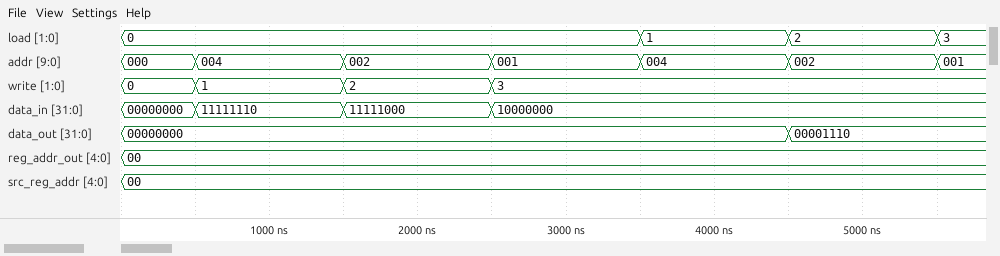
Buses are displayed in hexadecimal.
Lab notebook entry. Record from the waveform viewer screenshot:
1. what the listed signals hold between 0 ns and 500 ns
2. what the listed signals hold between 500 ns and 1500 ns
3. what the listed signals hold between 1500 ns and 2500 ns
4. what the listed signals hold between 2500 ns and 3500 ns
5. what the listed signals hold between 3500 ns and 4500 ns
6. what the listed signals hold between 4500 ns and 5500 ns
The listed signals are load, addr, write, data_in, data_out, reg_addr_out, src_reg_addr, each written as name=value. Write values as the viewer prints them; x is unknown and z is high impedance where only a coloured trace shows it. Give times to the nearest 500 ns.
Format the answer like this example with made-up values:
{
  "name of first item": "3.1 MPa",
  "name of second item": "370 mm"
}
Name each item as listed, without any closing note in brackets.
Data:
{
  "what the listed signals hold between 0 ns and 500 ns": "load=0, addr=000, write=0, data_in=00000000, data_out=00000000, reg_addr_out=00, src_reg_addr=00",
  "what the listed signals hold between 500 ns and 1500 ns": "load=0, addr=004, write=1, data_in=11111110, data_out=00000000, reg_addr_out=00, src_reg_addr=00",
  "what the listed signals hold between 1500 ns and 2500 ns": "load=0, addr=002, write=2, data_in=11111000, data_out=00000000, reg_addr_out=00, src_reg_addr=00",
  "what the listed signals hold between 2500 ns and 3500 ns": "load=0, addr=001, write=3, data_in=10000000, data_out=00000000, reg_addr_out=00, src_reg_addr=00",
  "what the listed signals hold between 3500 ns and 4500 ns": "load=1, addr=004, write=3, data_in=10000000, data_out=00000000, reg_addr_out=00, src_reg_addr=00",
  "what the listed signals hold between 4500 ns and 5500 ns": "load=2, addr=002, write=3, data_in=10000000, data_out=00001110, reg_addr_out=00, src_reg_addr=00"
}
